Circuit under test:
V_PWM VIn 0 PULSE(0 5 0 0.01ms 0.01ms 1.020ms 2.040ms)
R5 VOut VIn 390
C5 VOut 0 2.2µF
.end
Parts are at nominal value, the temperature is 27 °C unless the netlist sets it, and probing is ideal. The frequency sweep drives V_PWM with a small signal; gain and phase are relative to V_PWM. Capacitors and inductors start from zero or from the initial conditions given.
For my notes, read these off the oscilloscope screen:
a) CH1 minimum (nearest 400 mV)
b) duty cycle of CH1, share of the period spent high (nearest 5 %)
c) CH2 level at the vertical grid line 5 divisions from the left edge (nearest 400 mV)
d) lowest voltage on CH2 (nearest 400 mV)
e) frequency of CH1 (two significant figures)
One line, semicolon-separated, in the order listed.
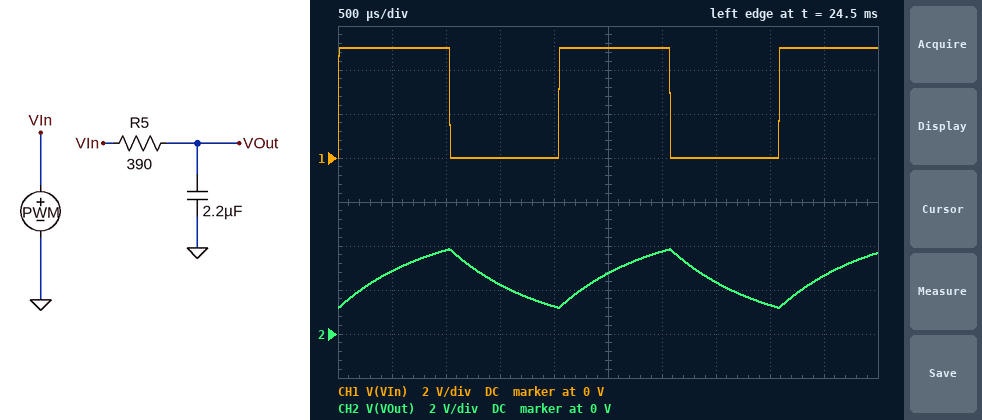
0 V; 50 %; 2.8 V; 1.2 V; 490 Hz
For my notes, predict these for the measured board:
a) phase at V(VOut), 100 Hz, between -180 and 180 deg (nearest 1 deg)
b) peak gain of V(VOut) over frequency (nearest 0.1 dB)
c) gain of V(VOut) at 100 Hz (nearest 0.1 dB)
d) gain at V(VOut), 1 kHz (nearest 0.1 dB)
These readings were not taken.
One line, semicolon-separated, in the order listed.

-28 deg; 0 dB; -1.1 dB; -14.8 dB
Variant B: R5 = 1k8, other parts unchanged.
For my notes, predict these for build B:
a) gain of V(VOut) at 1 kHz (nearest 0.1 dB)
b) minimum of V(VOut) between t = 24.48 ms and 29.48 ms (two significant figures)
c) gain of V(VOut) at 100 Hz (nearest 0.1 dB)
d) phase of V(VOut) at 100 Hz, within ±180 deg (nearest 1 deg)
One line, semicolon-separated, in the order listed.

-27.9 dB; 2.2 V; -8.6 dB; -68 deg
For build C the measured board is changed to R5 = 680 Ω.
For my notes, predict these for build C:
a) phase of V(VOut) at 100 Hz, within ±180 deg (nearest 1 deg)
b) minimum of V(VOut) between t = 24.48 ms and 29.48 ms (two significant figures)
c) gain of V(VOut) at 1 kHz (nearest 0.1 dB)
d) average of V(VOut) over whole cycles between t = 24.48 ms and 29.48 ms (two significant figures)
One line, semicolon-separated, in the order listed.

-43 deg; 1.7 V; -19.5 dB; 2.5 V
